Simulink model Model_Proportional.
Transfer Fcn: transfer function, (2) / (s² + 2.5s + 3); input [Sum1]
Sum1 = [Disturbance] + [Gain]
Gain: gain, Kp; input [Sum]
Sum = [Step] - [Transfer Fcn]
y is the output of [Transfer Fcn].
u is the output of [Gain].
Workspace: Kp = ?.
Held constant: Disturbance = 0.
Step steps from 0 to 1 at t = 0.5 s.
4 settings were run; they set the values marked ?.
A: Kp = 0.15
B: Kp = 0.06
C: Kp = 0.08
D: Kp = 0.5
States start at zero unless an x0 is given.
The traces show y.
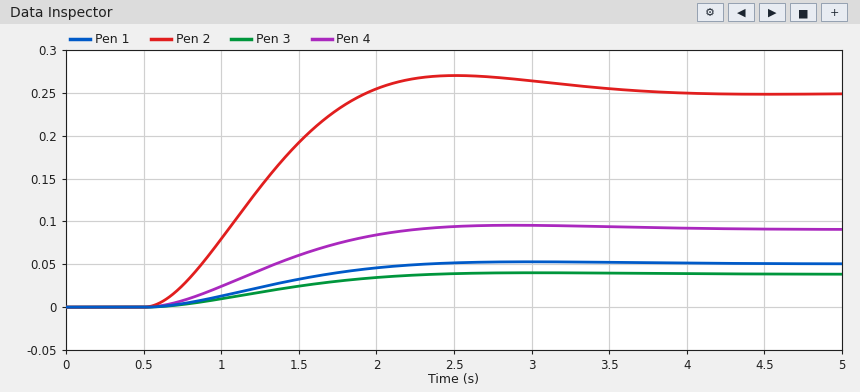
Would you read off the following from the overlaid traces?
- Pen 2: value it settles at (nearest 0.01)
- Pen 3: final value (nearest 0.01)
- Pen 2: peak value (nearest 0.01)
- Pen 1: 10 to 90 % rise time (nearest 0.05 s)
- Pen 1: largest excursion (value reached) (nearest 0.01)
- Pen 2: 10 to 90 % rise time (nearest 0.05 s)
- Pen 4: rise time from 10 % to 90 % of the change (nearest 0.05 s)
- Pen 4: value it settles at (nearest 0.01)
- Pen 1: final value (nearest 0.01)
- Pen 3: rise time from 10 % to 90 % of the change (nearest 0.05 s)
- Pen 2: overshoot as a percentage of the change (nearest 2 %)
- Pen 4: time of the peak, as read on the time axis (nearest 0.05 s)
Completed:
0.25
0.04
0.27
1.20 s
0.05
0.95 s
1.15 s
0.09
0.05
1.20 s
8 %
2.90 s
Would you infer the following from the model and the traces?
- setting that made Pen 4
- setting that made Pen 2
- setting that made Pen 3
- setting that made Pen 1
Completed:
A
D
B
C
